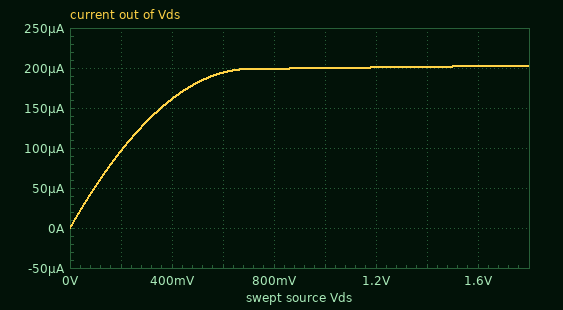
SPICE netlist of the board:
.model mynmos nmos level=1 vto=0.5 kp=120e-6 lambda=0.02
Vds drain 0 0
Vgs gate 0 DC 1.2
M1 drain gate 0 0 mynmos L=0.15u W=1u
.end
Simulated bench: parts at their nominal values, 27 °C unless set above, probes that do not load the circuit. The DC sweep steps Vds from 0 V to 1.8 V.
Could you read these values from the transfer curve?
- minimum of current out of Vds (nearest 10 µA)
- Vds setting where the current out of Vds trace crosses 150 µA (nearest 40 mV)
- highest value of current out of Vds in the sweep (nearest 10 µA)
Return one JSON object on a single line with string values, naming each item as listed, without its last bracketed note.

{"minimum of current out of Vds": "0 A", "Vds setting where the current out of Vds trace crosses 150 µA": "360 mV", "highest value of current out of Vds in the sweep": "200 µA"}
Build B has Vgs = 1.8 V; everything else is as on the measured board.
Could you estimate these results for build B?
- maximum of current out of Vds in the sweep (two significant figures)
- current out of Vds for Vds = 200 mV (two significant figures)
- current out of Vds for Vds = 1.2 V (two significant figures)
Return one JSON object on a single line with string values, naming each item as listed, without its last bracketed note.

{"maximum of current out of Vds in the sweep": "700 µA", "current out of Vds for Vds = 200 mV": "190 µA", "current out of Vds for Vds = 1.2 V": "690 µA"}
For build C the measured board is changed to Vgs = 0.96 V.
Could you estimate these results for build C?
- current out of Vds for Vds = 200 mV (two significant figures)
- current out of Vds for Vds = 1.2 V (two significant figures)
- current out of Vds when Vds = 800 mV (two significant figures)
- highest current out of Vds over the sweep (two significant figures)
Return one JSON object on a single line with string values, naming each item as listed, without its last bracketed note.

{"current out of Vds for Vds = 200 mV": "58 µA", "current out of Vds for Vds = 1.2 V": "87 µA", "current out of Vds when Vds = 800 mV": "86 µA", "highest current out of Vds over the sweep": "88 µA"}
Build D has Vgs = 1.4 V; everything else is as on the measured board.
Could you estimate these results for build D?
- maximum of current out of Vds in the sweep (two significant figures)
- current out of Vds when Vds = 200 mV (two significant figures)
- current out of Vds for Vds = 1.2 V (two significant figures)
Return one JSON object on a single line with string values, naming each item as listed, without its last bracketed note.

{"maximum of current out of Vds in the sweep": "340 µA", "current out of Vds when Vds = 200 mV": "130 µA", "current out of Vds for Vds = 1.2 V": "330 µA"}
